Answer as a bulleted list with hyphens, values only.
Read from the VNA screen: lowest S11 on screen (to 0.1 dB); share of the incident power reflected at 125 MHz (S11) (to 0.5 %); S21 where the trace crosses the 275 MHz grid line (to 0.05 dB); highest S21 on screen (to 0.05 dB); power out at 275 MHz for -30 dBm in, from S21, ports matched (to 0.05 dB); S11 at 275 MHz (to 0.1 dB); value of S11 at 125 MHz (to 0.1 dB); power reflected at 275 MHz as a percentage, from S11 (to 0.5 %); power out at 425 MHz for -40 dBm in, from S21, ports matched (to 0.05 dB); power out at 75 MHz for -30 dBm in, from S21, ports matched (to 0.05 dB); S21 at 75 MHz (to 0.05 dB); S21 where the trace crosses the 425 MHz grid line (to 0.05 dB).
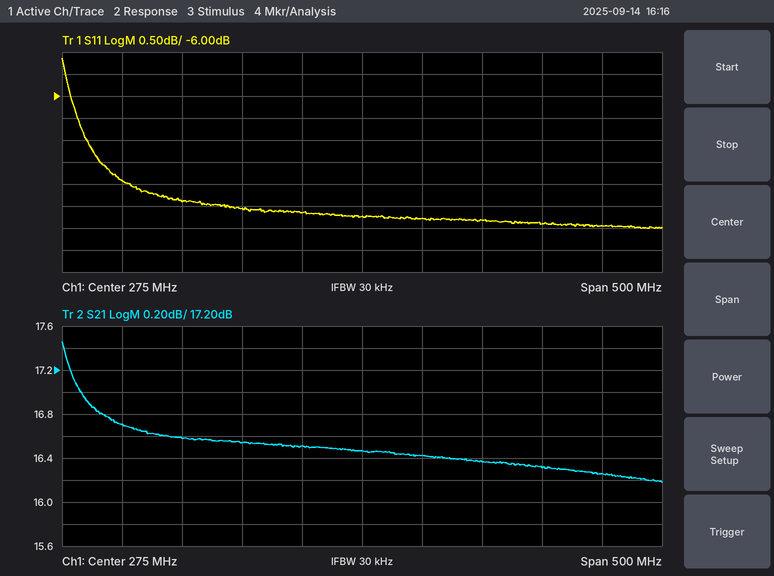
- -9.0 dB
- 14.5 %
- 16.45 dB
- 17.45 dB
- -13.55 dBm
- -8.7 dB
- -8.4 dB
- 13.5 %
- -23.70 dBm
- -13.30 dBm
- 16.70 dB
- 16.30 dB
